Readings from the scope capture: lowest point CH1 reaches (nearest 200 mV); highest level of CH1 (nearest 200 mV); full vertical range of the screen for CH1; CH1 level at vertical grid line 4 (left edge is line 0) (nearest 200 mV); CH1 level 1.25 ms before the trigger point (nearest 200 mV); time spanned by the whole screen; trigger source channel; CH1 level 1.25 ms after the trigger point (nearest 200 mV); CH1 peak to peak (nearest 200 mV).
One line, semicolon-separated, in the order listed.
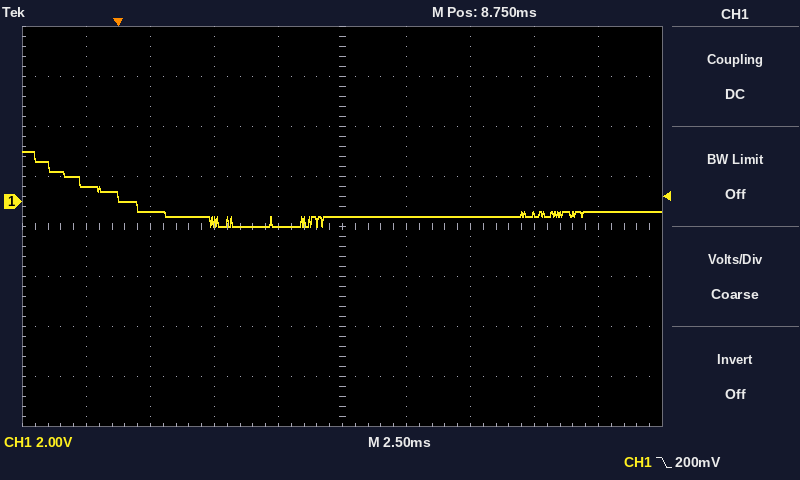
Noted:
-1.0 V; 2.0 V; 16 V; -1.0 V; 600 mV; 25 ms; CH1; -400 mV; 3.0 V
